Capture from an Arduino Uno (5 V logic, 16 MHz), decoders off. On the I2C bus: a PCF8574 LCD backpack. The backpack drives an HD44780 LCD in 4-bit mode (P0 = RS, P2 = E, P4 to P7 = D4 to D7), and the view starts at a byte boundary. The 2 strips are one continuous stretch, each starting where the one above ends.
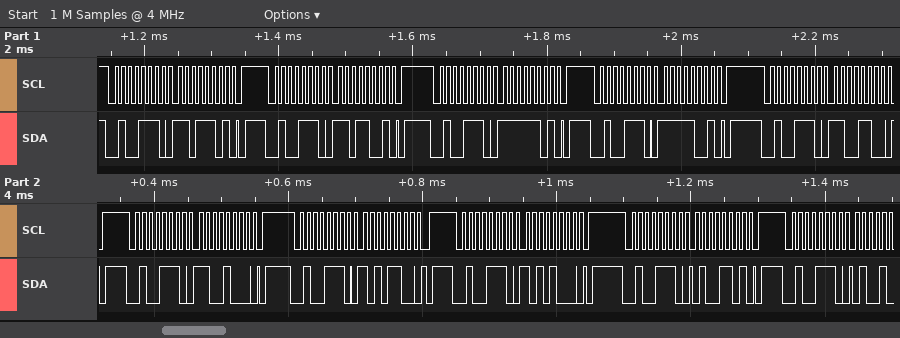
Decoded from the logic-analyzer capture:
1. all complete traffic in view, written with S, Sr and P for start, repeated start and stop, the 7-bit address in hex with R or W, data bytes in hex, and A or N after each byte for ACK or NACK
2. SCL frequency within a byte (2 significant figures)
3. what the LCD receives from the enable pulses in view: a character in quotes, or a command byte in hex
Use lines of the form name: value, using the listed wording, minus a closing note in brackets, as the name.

all complete traffic in view, written with S, Sr and P for start, repeated start and stop, the 7-bit address in hex with R or W, data bytes in hex, and A or N after each byte for ACK or NACK: S 27W A DD A P S 27W A D9 A P S 27W A FD A P S 27W A F9 A P S 27W A CC A P S 27W A C8 A P S 27W A AC A P S 27W A A8 A P S 27W A 4D A P S 27W A
SCL frequency within a byte: 100 kHz
what the LCD receives from the enable pulses in view: a character in quotes, or a command byte in hex: data 0xDF 0xCA
